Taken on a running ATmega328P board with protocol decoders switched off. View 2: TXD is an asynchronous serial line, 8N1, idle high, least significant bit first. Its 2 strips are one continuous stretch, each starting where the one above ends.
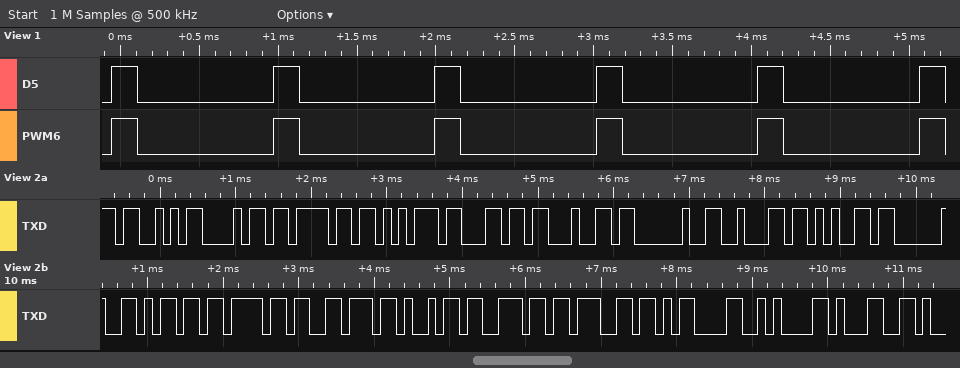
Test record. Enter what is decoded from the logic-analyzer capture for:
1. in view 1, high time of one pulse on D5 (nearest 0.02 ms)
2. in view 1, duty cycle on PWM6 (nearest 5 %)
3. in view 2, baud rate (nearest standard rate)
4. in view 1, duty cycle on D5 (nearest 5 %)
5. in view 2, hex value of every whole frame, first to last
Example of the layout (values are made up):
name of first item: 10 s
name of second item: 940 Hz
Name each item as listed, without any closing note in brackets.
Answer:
in view 1, high time of one pulse on D5: 0.16 ms
in view 1, duty cycle on PWM6: 15 %
in view 2, baud rate: 9600 baud
in view 1, duty cycle on D5: 15 %
in view 2, hex value of every whole frame, first to last: 53 68 6F 75 6C 64 20 62 65 20 6D 6F 76 69 6E 67 0D 0A 31
